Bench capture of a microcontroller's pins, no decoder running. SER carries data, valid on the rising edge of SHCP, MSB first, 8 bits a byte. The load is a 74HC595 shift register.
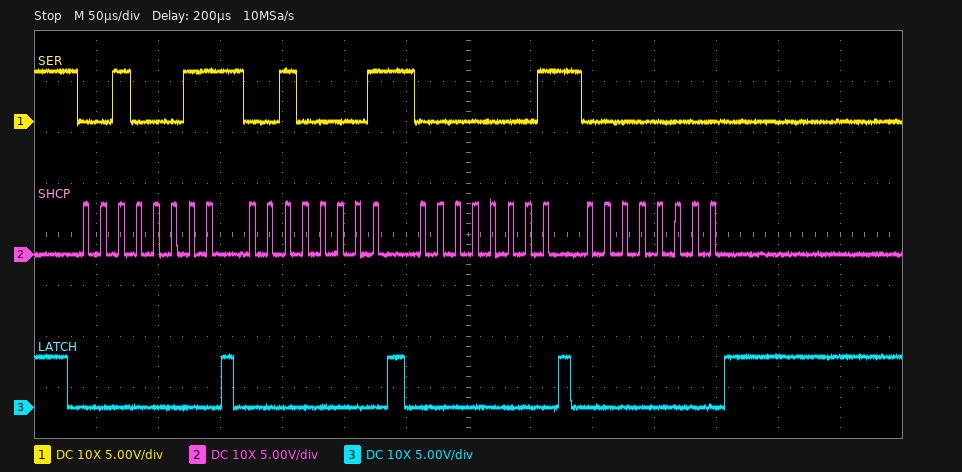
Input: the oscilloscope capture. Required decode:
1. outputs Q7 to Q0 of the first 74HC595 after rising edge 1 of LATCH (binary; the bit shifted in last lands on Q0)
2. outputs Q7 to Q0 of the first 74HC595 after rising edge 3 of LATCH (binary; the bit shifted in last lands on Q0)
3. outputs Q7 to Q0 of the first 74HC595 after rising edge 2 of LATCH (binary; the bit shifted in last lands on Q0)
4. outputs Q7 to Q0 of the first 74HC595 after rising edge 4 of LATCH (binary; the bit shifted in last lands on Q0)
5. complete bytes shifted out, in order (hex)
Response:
00100011
00000001
00100001
00000000
23 21 01 00
